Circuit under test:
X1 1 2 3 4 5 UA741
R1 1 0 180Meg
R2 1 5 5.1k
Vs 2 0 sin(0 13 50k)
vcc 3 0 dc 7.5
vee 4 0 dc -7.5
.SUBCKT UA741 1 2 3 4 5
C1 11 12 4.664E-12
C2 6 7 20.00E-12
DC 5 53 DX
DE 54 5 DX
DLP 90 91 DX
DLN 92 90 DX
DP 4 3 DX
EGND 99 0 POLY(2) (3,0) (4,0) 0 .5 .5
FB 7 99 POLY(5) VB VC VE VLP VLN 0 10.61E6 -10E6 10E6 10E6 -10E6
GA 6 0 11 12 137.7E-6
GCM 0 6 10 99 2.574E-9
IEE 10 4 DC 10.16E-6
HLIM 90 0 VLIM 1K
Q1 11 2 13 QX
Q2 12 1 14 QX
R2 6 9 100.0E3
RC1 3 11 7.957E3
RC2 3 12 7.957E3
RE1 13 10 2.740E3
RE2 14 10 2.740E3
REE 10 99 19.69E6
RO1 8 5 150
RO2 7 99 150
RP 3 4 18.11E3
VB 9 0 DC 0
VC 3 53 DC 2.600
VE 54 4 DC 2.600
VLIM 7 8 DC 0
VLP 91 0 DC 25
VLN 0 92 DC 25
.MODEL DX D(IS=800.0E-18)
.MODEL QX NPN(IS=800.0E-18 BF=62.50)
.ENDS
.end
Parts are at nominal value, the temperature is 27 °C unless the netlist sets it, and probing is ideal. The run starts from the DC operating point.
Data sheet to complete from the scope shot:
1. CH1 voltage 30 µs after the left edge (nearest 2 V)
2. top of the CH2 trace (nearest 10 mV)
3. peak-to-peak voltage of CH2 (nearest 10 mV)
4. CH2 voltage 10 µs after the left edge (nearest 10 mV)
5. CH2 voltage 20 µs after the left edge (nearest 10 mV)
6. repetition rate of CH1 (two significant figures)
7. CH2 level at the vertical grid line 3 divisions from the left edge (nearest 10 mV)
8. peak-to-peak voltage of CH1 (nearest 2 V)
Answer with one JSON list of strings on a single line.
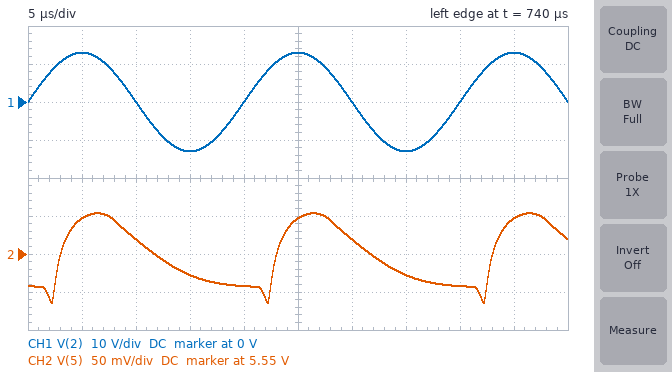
["0 V", "5.60 V", "120 mV", "5.57 V", "5.51 V", "50 kHz", "5.52 V", "26 V"]
